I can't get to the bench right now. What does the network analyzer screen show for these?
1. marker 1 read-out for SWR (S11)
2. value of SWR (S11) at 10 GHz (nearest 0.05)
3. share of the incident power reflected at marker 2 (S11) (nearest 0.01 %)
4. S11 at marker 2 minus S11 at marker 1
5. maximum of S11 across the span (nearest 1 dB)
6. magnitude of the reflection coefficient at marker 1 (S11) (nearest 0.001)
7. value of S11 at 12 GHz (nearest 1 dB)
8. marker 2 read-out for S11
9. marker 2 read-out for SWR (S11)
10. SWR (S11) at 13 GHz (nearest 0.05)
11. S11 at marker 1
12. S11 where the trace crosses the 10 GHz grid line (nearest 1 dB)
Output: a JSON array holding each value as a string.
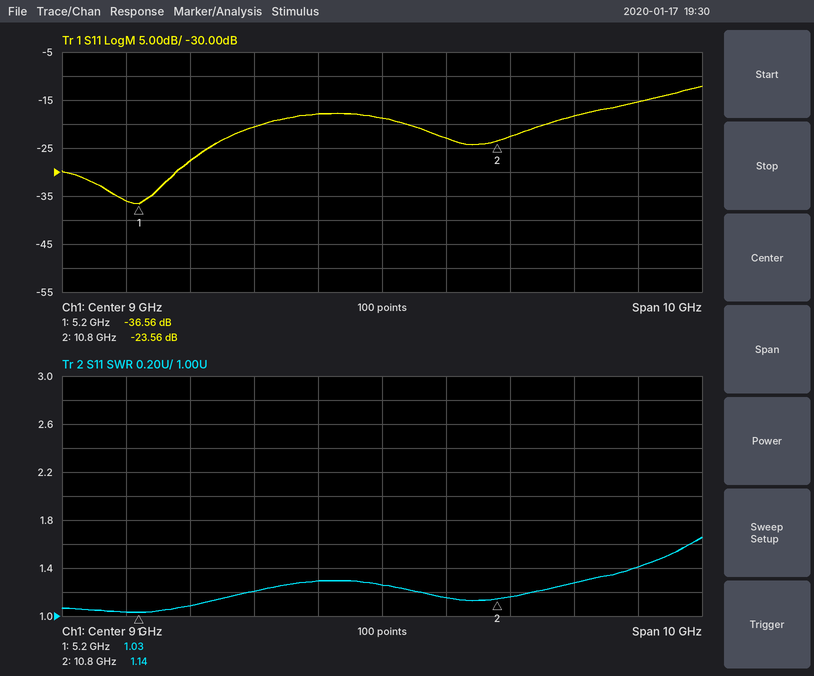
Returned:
["1.03", "1.15", "0.44 %", "13.00 dB", "-12 dB", "0.015", "-18 dB", "-23.56 dB", "1.14", "1.40", "-36.56 dB", "-23 dB"]
